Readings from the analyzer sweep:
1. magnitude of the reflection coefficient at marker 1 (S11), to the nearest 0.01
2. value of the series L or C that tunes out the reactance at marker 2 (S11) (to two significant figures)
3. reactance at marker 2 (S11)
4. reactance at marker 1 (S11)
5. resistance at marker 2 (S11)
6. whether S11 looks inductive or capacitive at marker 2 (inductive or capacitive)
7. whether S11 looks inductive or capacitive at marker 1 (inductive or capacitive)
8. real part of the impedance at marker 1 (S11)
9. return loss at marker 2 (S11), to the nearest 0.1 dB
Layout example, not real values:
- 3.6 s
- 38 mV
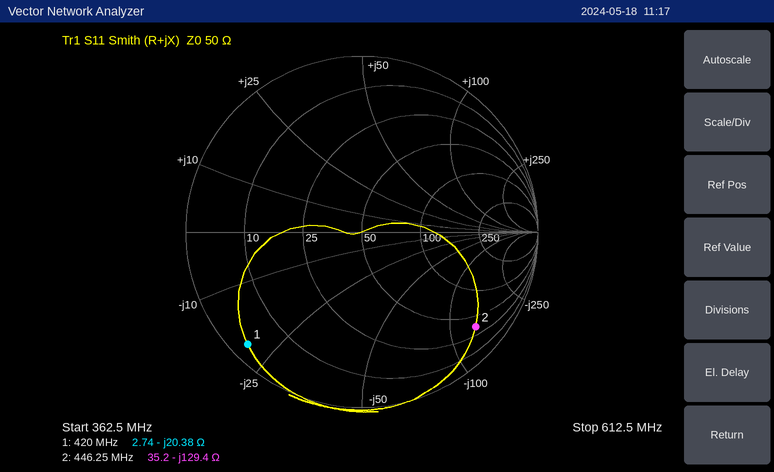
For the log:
- 0.91
- 46 nH
- -129.4 Ω
- -20.38 Ω
- 35.2 Ω
- capacitive
- capacitive
- 2.74 Ω
- 1.5 dB
